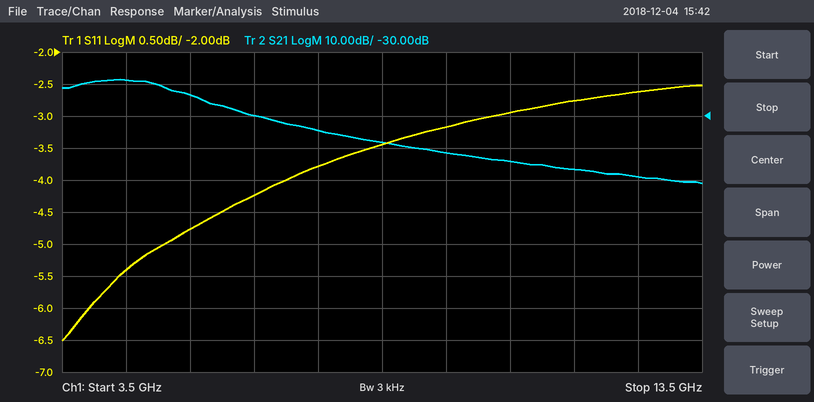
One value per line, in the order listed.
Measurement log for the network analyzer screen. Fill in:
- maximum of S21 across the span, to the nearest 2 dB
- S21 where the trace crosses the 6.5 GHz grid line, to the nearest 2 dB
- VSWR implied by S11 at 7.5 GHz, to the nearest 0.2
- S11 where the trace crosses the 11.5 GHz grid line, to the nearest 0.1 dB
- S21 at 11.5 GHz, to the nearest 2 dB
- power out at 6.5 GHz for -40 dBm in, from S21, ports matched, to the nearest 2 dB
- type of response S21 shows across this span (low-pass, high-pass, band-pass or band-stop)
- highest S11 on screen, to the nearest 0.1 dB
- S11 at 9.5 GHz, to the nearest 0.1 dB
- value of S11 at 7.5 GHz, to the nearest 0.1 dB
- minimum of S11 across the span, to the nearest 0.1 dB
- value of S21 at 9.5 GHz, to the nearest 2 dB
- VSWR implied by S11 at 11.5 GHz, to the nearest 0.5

-18 dB
-30 dB
4.6
-2.8 dB
-46 dB
-70 dBm
low-pass
-2.5 dB
-3.2 dB
-3.8 dB
-6.5 dB
-42 dB
6.5
